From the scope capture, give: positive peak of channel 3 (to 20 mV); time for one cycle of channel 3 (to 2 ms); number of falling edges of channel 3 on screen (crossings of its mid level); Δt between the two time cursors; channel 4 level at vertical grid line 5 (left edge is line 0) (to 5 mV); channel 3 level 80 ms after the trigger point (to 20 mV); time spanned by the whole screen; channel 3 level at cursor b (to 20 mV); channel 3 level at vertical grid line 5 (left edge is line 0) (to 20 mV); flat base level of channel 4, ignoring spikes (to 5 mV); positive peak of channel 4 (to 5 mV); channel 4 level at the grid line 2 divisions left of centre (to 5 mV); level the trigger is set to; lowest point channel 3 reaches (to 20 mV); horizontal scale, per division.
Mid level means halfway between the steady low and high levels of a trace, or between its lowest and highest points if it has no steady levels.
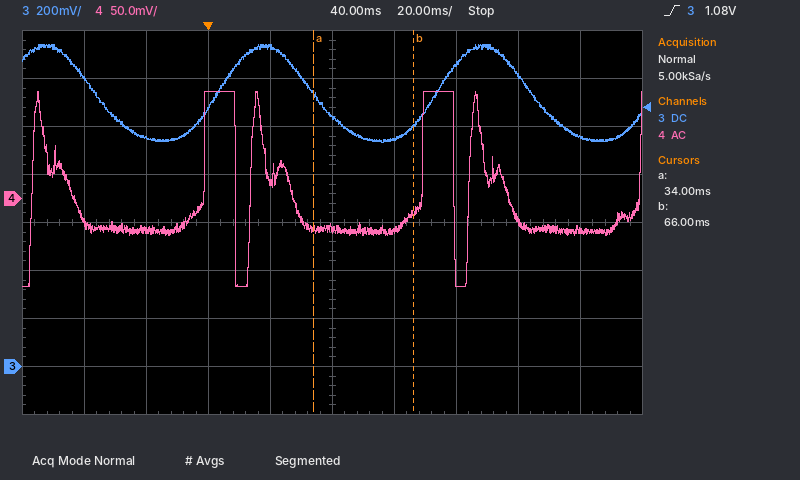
1.34 V
70 ms
3
32 ms
-30 mV
1.26 V
200 ms
1.00 V
1.04 V
-35 mV
110 mV
110 mV
1.08 V
940 mV
20 ms
